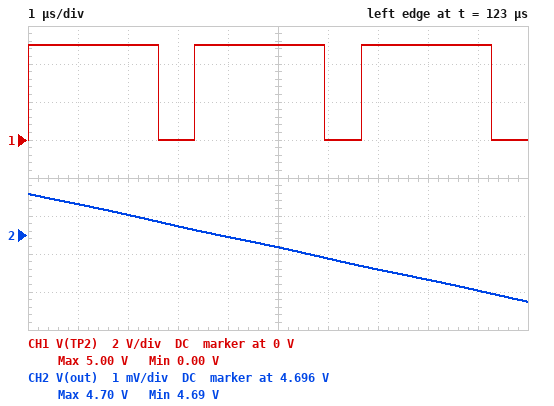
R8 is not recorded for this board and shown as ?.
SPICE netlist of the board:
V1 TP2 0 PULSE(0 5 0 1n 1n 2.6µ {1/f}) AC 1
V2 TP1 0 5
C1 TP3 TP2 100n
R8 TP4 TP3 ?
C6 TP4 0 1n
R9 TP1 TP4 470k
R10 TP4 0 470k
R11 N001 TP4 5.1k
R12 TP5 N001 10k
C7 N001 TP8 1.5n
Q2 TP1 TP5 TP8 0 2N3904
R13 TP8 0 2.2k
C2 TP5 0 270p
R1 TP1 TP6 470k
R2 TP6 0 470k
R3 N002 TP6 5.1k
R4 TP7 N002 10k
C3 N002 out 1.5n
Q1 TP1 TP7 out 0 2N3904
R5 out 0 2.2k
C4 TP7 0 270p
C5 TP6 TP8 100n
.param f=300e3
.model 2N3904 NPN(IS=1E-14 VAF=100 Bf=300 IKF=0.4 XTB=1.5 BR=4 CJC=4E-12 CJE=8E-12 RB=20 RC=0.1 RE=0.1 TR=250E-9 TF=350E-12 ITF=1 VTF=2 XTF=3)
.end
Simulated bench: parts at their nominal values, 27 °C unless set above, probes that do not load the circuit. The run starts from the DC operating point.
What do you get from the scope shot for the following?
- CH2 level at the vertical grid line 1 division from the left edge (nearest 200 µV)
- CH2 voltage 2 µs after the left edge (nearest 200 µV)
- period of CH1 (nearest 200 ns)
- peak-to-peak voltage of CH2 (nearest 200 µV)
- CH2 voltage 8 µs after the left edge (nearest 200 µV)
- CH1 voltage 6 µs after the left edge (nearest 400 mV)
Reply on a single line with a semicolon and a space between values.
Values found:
4.6968 V; 4.6966 V; 3.4 µs; 2.8 mV; 4.6948 V; 0 V
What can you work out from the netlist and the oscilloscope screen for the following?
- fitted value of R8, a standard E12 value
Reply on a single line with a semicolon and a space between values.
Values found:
10 kΩ
